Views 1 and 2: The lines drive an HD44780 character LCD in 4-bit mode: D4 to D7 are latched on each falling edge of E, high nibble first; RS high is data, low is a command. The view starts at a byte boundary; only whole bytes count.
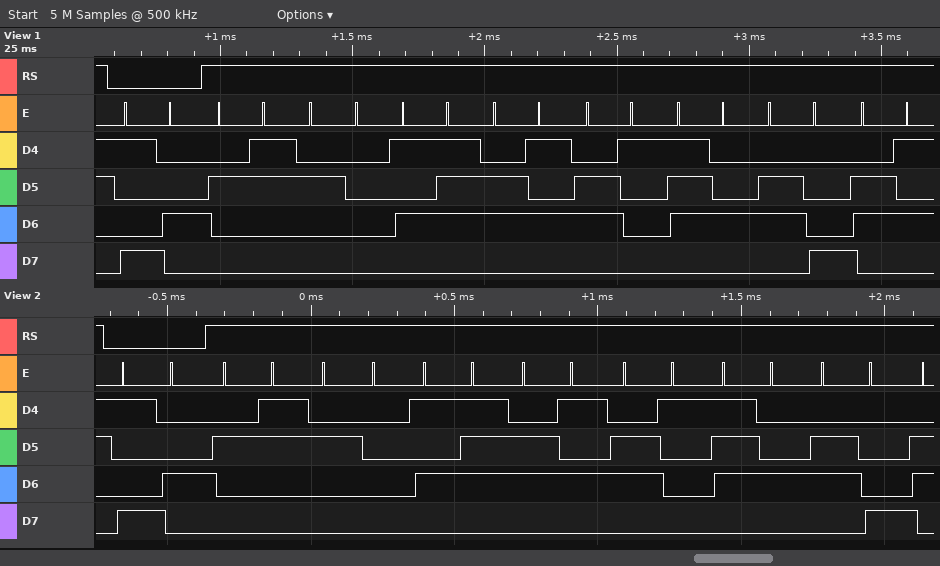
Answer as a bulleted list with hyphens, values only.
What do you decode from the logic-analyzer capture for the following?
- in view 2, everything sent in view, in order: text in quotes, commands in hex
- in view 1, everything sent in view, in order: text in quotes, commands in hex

- 0x94 "# Weath"
- 0x94 "# Weathe"
